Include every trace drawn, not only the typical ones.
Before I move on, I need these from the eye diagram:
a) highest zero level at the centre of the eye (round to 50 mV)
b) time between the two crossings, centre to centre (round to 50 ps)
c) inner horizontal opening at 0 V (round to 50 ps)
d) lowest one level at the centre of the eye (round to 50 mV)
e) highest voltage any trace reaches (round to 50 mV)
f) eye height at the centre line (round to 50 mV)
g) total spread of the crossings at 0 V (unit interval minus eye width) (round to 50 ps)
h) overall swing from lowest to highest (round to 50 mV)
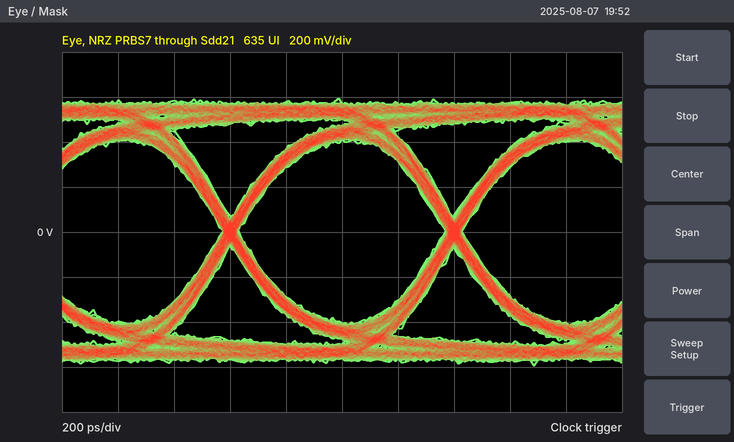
-400 mV
800 ps
750 ps
400 mV
600 mV
800 mV
50 ps
1.20 V
